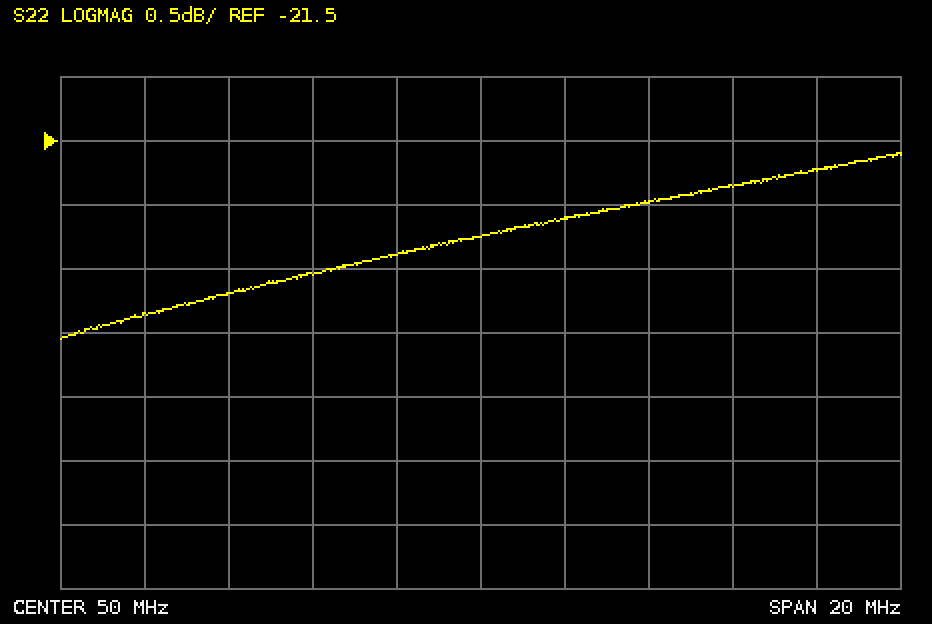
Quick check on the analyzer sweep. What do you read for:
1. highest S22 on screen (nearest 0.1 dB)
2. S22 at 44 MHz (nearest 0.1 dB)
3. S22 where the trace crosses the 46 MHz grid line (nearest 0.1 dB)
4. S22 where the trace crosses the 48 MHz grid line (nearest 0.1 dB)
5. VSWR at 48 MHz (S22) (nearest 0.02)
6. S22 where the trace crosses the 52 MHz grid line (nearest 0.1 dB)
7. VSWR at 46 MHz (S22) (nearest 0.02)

-21.6 dB
-22.7 dB
-22.5 dB
-22.4 dB
1.16
-22.1 dB
1.16
